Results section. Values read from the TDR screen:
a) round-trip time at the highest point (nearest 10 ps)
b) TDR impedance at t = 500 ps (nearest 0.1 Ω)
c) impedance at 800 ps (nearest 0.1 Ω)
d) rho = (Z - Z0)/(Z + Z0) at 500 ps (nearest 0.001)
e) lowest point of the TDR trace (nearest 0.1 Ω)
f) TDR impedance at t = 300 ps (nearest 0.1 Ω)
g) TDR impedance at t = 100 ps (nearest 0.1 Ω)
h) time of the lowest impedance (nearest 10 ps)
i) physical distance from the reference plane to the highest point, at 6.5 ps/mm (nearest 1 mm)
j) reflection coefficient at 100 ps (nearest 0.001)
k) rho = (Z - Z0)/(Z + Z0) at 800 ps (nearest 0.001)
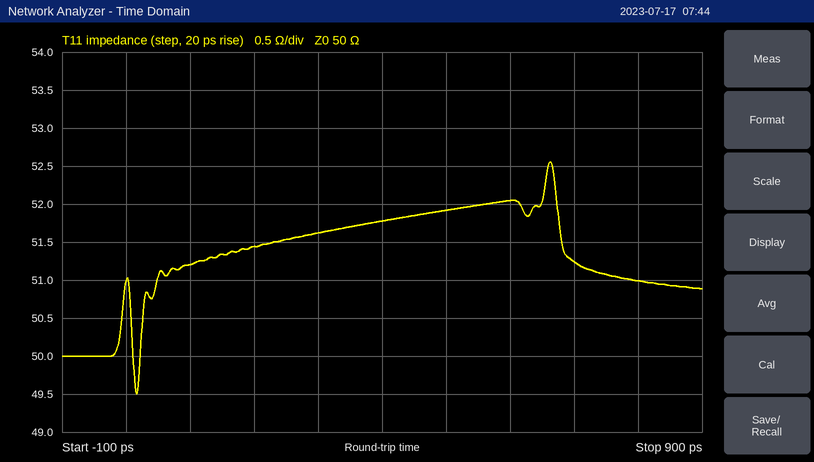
660 ps
51.9 Ω
51.0 Ω
+0.019
49.5 Ω
51.6 Ω
51.2 Ω
20 ps
51 mm
+0.012
+0.010
